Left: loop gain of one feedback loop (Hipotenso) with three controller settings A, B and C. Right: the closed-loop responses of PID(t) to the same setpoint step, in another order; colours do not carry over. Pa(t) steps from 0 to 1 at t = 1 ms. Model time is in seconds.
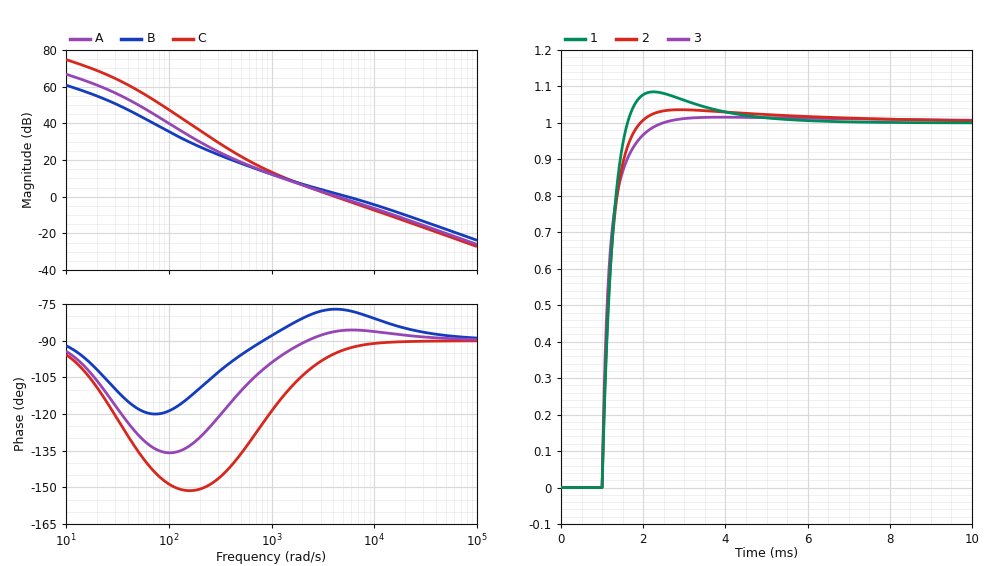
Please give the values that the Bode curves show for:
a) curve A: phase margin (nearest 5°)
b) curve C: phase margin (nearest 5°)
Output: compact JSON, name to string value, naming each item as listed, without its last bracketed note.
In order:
{"curve A: phase margin": "95°", "curve C: phase margin": "85°"}
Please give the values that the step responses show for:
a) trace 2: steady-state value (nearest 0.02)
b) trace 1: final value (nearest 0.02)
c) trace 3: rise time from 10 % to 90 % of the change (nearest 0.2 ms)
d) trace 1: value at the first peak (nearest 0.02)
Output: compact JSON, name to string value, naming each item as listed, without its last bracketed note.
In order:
{"trace 2: steady-state value": "1.00", "trace 1: final value": "1.00", "trace 3: rise time from 10 % to 90 % of the change": "0.6 ms", "trace 1: value at the first peak": "1.08"}
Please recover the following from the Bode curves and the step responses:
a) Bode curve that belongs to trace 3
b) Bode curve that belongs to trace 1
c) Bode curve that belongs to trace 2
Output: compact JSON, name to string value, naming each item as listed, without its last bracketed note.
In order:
{"Bode curve that belongs to trace 3": "B", "Bode curve that belongs to trace 1": "C", "Bode curve that belongs to trace 2": "A"}
